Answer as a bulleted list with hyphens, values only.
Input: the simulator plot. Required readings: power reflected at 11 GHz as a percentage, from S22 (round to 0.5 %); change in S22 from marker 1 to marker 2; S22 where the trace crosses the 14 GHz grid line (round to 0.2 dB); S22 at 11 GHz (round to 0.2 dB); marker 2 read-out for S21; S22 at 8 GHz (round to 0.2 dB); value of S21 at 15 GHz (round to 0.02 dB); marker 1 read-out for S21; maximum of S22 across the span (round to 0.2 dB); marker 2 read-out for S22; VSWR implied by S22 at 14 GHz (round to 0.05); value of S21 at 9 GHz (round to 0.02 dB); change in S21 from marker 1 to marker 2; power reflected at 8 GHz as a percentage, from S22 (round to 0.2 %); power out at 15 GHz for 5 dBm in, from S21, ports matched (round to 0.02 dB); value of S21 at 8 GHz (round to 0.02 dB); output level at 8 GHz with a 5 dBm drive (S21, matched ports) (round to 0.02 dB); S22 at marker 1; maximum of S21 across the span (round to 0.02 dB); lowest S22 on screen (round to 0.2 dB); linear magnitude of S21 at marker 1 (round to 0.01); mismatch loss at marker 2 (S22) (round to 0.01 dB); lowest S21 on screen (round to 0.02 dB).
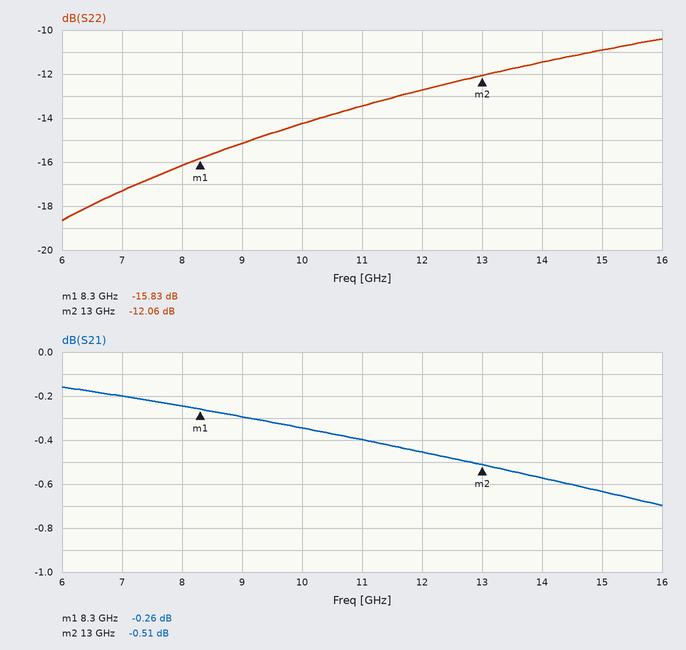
- 4.5 %
- 3.77 dB
- -11.4 dB
- -13.4 dB
- -0.51 dB
- -16.2 dB
- -0.64 dB
- -0.26 dB
- -10.4 dB
- -12.06 dB
- 1.75
- -0.30 dB
- -0.25 dB
- 2.4 %
- 4.36 dBm
- -0.24 dB
- 4.76 dBm
- -15.83 dB
- -0.16 dB
- -18.6 dB
- 0.97
- 0.28 dB
- -0.70 dB
